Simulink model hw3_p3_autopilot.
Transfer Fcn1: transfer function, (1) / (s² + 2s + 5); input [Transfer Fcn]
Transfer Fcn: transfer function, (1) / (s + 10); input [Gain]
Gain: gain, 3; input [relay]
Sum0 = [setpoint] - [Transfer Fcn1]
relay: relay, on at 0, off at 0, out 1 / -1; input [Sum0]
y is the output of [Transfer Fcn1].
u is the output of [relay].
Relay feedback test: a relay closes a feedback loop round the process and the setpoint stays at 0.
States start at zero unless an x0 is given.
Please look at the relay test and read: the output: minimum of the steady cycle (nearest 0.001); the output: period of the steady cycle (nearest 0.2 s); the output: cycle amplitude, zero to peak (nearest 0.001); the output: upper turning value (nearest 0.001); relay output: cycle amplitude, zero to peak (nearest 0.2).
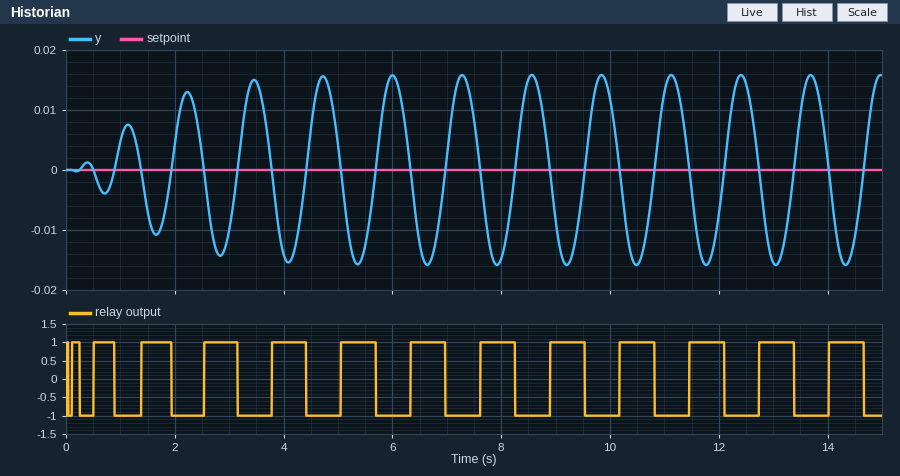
-0.016
1.2 s
0.016
0.016
1.0
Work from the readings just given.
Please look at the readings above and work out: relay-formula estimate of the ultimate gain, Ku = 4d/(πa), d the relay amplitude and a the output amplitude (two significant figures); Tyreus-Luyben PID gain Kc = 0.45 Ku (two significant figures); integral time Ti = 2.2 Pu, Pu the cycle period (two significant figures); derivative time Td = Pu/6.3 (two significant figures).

80
36
2.6 s
0.19 s
